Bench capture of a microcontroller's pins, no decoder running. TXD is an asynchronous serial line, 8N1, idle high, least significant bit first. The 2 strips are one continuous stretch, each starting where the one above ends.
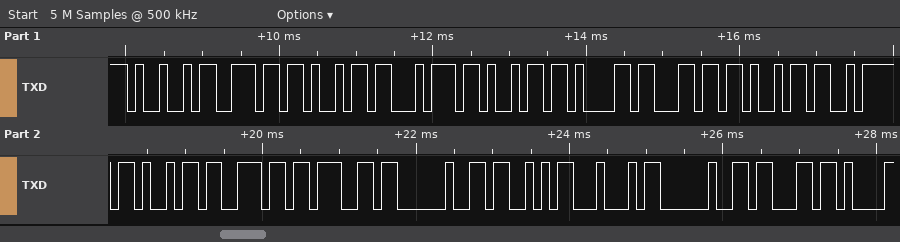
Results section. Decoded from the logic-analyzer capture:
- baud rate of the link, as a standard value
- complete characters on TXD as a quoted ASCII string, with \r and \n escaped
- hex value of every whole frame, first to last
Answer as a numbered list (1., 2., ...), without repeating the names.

1. 9600 baud
2. "Initializing SD c"
3. 49 6E 69 74 69 61 6C 69 7A 69 6E 67 20 53 44 20 63
